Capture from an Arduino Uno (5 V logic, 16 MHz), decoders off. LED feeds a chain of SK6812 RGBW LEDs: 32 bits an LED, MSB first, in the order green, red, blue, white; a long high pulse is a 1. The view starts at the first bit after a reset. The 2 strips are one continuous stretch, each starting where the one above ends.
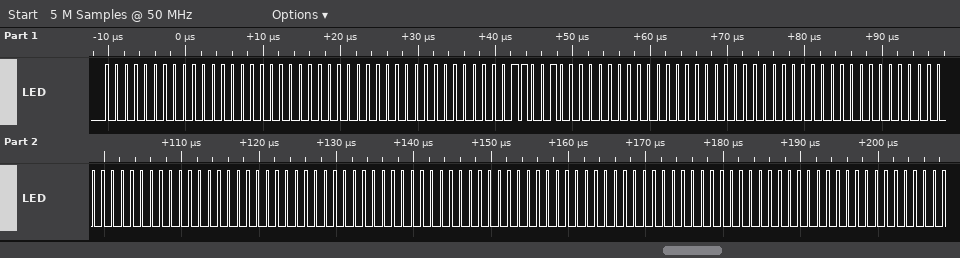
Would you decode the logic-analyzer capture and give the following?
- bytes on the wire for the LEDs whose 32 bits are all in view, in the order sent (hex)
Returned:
00 00 00 00 00 32 00 00 00 00 00 00 00 00 00 00 00 00 00 00
